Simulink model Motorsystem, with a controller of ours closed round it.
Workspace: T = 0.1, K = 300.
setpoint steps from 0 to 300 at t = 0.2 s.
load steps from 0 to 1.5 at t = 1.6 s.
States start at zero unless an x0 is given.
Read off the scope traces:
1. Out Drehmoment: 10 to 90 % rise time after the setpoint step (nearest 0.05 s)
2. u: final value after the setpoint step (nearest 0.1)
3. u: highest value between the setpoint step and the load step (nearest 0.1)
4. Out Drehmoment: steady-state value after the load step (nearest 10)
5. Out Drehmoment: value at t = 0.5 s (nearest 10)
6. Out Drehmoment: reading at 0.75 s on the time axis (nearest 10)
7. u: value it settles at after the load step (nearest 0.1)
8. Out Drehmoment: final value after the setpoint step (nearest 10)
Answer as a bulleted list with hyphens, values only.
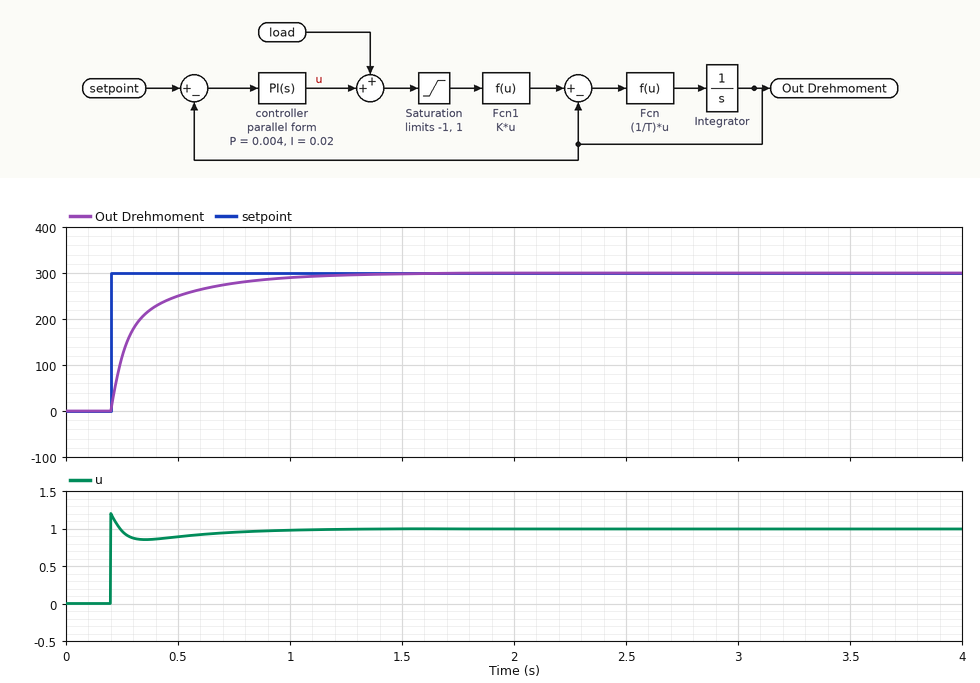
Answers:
- 0.45 s
- 1.0
- 1.2
- 300
- 250
- 280
- 1.0
- 300
